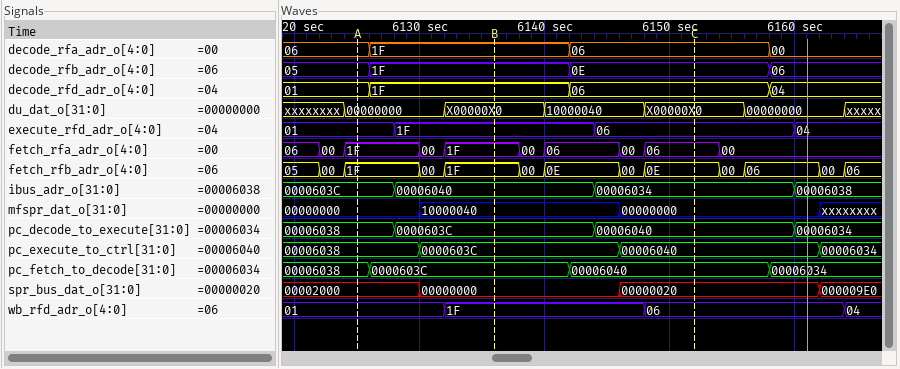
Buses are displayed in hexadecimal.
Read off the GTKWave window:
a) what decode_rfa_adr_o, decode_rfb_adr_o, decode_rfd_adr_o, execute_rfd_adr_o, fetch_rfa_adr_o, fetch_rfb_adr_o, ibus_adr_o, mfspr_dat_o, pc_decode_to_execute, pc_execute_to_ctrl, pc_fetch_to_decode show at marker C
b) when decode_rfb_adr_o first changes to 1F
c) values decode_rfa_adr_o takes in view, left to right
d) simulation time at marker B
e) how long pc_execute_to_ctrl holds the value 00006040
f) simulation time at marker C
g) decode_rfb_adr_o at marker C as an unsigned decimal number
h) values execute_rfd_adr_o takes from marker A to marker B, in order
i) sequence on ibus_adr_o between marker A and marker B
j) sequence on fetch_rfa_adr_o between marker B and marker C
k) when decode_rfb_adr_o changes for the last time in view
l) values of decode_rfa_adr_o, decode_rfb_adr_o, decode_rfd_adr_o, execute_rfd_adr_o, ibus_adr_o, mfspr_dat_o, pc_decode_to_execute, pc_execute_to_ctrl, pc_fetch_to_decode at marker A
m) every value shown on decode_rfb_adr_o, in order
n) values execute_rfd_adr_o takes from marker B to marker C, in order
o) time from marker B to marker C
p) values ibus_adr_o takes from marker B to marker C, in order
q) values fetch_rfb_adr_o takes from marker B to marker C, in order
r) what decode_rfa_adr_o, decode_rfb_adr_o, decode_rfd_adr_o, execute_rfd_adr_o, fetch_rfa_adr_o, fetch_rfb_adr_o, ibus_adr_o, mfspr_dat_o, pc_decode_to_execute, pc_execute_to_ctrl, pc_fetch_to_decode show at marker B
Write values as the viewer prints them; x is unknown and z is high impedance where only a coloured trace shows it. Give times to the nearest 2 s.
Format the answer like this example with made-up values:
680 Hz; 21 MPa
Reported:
decode_rfa_adr_o=06, decode_rfb_adr_o=0E, decode_rfd_adr_o=06, execute_rfd_adr_o=06, fetch_rfa_adr_o=06, fetch_rfb_adr_o=0E, ibus_adr_o=00006034, mfspr_dat_o=00000000, pc_decode_to_execute=00006040, pc_execute_to_ctrl=00006040, pc_fetch_to_decode=00006040; 6126 s; 06, 1F, 06, 00; 6136 s; 16 s; 6152 s; 14; 01, 1F; 0000603C, 00006040; 1F, 00, 06, 00, 06; 6158 s; decode_rfa_adr_o=06, decode_rfb_adr_o=05, decode_rfd_adr_o=01, execute_rfd_adr_o=01, ibus_adr_o=0000603C, mfspr_dat_o=00000000, pc_decode_to_execute=00006038, pc_execute_to_ctrl=00006038, pc_fetch_to_decode=00006038; 05, 1F, 0E, 06; 1F, 06; 16 s; 00006040, 00006034; 1F, 00, 0E, 00, 0E; decode_rfa_adr_o=1F, decode_rfb_adr_o=1F, decode_rfd_adr_o=1F, execute_rfd_adr_o=1F, fetch_rfa_adr_o=1F, fetch_rfb_adr_o=1F, ibus_adr_o=00006040, mfspr_dat_o=10000040, pc_decode_to_execute=0000603C, pc_execute_to_ctrl=0000603C, pc_fetch_to_decode=0000603C
